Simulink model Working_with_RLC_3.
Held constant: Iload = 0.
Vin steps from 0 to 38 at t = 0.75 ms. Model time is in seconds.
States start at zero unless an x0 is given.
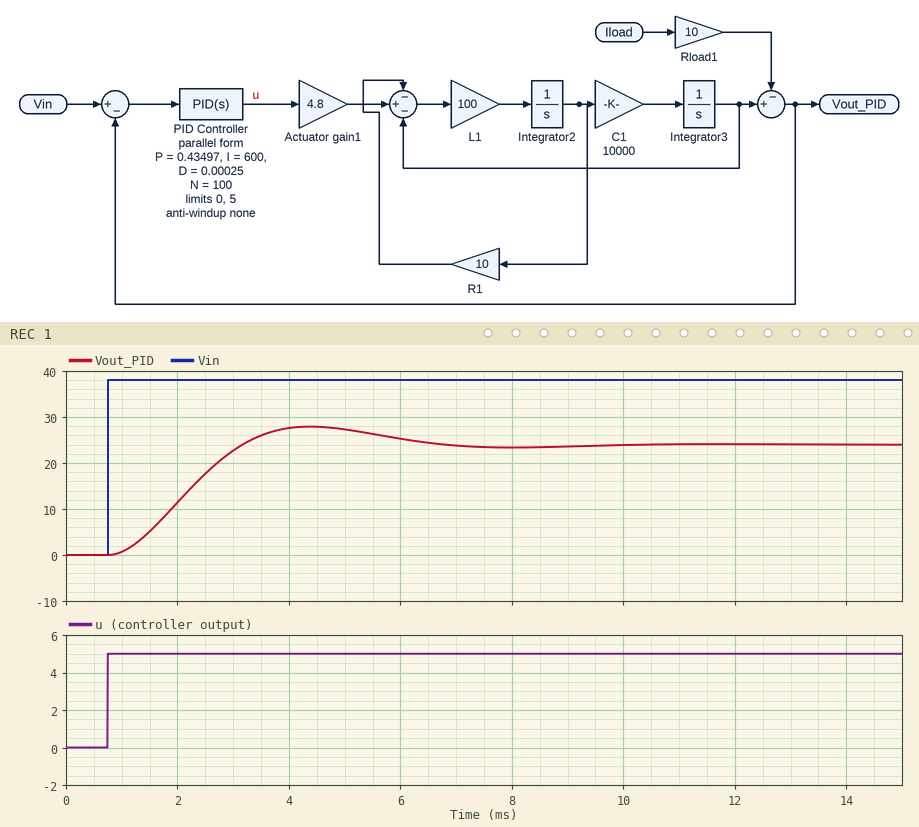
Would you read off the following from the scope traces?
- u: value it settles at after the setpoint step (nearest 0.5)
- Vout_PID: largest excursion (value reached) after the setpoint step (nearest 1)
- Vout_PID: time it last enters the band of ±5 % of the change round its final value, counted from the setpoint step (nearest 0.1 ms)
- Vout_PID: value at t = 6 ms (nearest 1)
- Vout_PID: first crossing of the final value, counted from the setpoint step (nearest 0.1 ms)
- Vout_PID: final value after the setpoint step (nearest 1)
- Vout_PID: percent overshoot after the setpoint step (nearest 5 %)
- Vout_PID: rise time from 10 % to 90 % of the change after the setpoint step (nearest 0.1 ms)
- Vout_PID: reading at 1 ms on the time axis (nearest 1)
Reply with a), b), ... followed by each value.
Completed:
a) 5.0
b) 28
c) 5.3 ms
d) 25
e) 2.4 ms
f) 24
g) 15 %
h) 1.6 ms
i) 1
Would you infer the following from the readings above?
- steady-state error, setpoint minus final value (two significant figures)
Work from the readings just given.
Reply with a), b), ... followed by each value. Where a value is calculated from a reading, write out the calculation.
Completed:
a) 38 - 24 = 14
